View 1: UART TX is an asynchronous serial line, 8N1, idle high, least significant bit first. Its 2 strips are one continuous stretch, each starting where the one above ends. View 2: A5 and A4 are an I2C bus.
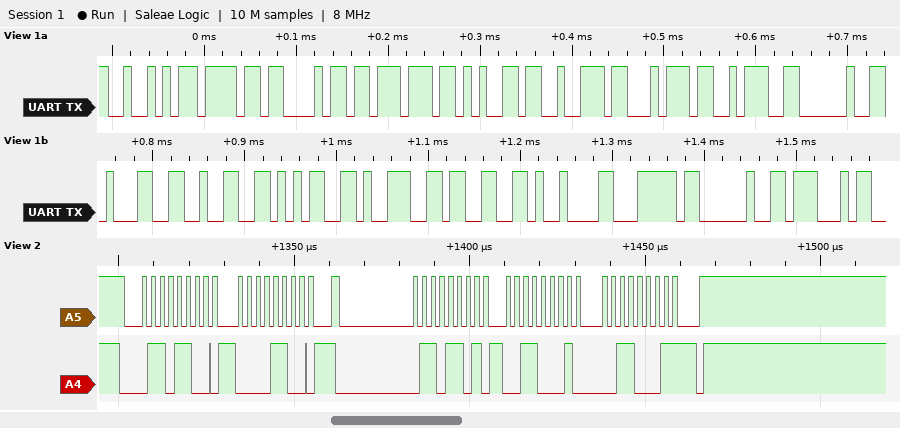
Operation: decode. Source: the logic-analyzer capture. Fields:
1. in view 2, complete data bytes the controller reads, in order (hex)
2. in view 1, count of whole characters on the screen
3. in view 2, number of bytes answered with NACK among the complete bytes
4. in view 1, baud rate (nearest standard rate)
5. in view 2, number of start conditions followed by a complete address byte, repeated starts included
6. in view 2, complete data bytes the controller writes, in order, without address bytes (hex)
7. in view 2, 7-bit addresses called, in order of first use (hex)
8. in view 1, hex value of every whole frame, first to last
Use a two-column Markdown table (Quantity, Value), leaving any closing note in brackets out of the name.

| Quantity | Value |
|---|---|
| in view 2, complete data bytes the controller reads, in order | 31 31 |
| in view 1, count of whole characters on the screen | 18 |
| in view 2, number of bytes answered with NACK among the complete bytes | 1 |
| in view 1, baud rate | 115200 baud |
| in view 2, number of start conditions followed by a complete address byte, repeated starts included | 2 |
| in view 2, complete data bytes the controller writes, in order, without address bytes | 0C |
| in view 2, 7-bit addresses called, in order of first use | 0x36 |
| in view 1, hex value of every whole frame, first to last | 0x52 0x6F 0x68 0x77 0x65 0x72 0x74 0x3A 0x20 0x31 0x32 0x35 0x39 0x33 0x09 0x7C 0x20 0x47 |
